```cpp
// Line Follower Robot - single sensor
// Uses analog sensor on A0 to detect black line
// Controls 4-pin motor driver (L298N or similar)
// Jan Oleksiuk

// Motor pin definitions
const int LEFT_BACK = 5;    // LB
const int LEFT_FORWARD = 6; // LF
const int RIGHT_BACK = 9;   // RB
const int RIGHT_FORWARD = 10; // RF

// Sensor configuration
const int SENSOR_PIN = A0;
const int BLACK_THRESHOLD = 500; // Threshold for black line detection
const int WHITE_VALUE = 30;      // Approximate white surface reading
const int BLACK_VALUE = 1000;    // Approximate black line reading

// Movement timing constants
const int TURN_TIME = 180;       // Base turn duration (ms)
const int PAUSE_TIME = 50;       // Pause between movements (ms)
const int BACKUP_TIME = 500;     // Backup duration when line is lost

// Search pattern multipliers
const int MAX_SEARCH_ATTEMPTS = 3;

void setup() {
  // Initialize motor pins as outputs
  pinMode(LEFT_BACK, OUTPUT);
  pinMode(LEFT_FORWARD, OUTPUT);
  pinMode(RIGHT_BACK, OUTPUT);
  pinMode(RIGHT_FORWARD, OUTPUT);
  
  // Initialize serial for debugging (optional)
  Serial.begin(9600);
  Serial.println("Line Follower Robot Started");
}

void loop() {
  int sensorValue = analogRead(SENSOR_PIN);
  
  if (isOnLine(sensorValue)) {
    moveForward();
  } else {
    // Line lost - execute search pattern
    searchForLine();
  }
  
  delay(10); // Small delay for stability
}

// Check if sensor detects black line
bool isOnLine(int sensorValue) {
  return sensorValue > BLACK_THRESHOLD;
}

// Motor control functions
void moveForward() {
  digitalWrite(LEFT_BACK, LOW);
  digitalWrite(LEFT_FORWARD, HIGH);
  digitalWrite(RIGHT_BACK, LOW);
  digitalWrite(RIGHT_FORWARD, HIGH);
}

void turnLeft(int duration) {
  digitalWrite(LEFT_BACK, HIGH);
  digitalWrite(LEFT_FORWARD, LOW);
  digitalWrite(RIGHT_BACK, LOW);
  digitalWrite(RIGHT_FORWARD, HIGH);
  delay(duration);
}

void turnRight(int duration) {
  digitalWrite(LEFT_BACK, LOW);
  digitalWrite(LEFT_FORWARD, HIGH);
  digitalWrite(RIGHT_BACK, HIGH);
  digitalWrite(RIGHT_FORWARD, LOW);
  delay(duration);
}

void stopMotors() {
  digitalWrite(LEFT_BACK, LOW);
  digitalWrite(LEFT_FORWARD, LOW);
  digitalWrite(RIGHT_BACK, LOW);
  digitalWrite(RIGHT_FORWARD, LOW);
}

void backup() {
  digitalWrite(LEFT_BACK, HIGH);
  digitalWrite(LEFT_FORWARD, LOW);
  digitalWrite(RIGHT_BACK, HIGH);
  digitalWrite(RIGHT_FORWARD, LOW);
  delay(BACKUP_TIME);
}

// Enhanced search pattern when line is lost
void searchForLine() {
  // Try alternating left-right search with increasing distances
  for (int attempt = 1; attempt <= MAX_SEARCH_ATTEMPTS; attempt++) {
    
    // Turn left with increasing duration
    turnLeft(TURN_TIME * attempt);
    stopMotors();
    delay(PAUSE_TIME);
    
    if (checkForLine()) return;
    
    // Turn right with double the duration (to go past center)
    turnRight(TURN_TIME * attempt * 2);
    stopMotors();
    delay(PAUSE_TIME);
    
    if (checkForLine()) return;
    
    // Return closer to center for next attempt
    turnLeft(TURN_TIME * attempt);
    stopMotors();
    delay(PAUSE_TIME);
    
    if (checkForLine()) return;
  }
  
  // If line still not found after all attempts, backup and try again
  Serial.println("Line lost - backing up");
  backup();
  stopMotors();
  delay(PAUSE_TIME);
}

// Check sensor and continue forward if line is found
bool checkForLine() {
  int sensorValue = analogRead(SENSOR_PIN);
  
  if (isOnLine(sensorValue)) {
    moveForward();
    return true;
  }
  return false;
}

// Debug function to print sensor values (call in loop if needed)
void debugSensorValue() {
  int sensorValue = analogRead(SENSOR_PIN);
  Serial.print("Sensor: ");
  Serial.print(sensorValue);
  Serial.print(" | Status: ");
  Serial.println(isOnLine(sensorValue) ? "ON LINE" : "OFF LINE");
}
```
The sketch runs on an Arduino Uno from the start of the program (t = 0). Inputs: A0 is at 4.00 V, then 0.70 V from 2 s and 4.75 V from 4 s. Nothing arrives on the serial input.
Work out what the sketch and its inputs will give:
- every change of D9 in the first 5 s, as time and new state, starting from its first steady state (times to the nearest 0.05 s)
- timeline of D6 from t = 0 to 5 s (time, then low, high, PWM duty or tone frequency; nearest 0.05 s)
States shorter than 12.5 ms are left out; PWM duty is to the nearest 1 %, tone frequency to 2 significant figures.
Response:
0 s low; 2.25 s high; 2.6 s low; 3.3 s high; 4 s low
0 s high; 2 s low; 2.25 s high; 2.6 s low; 3.3 s high; 4 s low; 4.05 s high
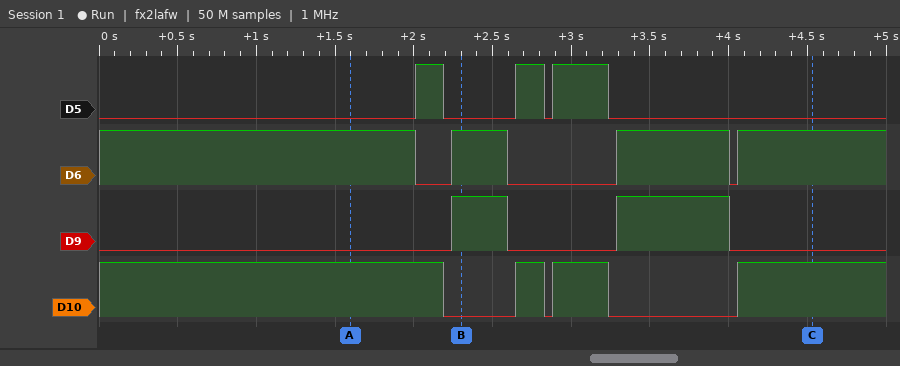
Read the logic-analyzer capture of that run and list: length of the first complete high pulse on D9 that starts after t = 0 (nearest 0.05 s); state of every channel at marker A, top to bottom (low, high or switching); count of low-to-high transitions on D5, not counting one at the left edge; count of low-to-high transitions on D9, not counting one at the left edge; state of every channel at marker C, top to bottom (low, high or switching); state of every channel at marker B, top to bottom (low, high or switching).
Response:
0.35 s
D5 low, D6 high, D9 low, D10 high
3
2
D5 low, D6 high, D9 low, D10 high
D5 low, D6 high, D9 high, D10 low
